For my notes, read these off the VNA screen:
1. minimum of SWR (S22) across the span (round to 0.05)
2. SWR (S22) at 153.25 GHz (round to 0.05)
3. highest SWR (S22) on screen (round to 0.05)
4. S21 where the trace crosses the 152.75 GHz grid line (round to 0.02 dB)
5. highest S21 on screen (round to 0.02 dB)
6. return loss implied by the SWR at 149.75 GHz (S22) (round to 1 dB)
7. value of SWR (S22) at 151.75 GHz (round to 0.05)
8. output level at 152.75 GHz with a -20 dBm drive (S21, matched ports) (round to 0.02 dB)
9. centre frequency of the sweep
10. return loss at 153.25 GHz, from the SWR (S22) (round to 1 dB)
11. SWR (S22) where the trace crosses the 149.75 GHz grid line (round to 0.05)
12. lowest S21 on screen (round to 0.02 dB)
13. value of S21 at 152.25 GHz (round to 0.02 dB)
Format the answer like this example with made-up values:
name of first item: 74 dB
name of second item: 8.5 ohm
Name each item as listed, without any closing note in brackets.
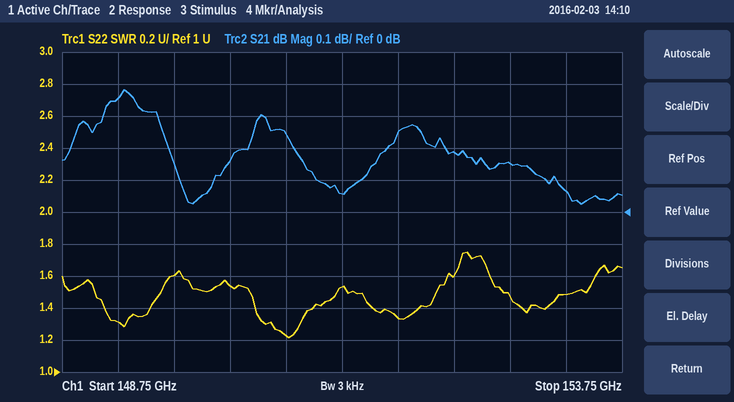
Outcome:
minimum of SWR (S22) across the span: 1.20
SWR (S22) at 153.25 GHz: 1.50
highest SWR (S22) on screen: 1.75
S21 where the trace crosses the 152.75 GHz grid line: 0.16 dB
highest S21 on screen: 0.38 dB
return loss implied by the SWR at 149.75 GHz (S22): 13 dB
value of SWR (S22) at 151.75 GHz: 1.35
output level at 152.75 GHz with a -20 dBm drive (S21, matched ports): -19.84 dBm
centre frequency of the sweep: 151.25 GHz
return loss at 153.25 GHz, from the SWR (S22): 14 dB
SWR (S22) where the trace crosses the 149.75 GHz grid line: 1.60
lowest S21 on screen: 0.02 dB
value of S21 at 152.25 GHz: 0.18 dB
